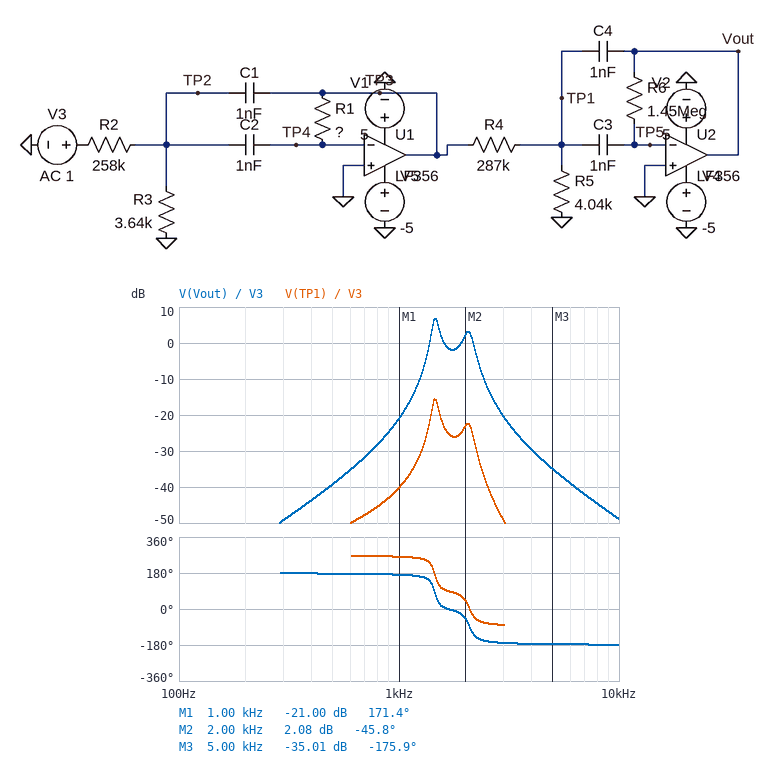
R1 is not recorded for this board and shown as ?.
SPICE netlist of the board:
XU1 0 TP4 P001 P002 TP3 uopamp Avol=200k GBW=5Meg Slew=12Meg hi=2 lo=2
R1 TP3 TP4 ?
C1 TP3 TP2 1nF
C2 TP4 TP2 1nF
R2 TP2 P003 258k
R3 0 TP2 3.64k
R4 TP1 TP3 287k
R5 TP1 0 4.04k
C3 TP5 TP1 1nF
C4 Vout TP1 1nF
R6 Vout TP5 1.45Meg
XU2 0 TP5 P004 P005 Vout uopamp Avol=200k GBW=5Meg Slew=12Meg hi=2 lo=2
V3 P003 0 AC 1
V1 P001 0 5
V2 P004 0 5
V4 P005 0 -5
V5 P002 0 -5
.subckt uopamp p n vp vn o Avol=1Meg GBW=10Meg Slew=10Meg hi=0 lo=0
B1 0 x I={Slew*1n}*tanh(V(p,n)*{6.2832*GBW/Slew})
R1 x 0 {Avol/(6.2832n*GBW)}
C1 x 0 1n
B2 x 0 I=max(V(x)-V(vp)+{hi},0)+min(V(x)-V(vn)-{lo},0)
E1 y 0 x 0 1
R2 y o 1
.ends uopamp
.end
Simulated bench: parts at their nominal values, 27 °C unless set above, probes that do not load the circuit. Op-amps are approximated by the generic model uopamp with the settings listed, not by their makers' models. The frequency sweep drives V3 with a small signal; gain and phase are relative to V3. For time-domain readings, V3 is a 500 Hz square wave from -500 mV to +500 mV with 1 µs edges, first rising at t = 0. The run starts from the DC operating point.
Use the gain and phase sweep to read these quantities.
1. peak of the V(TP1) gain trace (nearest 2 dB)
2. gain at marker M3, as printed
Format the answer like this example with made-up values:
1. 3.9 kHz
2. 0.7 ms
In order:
1. -16 dB
2. -35.01 dB
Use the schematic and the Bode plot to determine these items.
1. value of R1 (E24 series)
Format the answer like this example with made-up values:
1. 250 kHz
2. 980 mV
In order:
1. 3.3 MΩ
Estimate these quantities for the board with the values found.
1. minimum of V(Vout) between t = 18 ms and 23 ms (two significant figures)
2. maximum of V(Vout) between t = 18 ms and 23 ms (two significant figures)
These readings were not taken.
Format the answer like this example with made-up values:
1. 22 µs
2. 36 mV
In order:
1. -420 mV
2. 420 mV
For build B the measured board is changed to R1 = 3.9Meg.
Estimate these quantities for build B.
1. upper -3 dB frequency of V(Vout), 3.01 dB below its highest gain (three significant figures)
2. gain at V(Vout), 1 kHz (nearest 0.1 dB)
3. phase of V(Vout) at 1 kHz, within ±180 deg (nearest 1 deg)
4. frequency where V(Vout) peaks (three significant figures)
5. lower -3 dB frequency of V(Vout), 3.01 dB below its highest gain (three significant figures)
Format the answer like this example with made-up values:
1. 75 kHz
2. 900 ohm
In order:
1. 1.39 kHz
2. -18.0 dB
3. 170 deg
4. 1.34 kHz
5. 1.30 kHz
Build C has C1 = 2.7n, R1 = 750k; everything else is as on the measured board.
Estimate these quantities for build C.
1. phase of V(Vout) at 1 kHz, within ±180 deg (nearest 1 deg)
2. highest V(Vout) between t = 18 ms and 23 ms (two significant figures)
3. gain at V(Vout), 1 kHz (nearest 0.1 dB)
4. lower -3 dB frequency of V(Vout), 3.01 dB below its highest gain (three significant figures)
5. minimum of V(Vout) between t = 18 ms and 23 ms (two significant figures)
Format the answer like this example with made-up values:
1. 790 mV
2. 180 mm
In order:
1. 170 deg
2. 40 mV
3. -36.5 dB
4. 1.87 kHz
5. -40 mV
